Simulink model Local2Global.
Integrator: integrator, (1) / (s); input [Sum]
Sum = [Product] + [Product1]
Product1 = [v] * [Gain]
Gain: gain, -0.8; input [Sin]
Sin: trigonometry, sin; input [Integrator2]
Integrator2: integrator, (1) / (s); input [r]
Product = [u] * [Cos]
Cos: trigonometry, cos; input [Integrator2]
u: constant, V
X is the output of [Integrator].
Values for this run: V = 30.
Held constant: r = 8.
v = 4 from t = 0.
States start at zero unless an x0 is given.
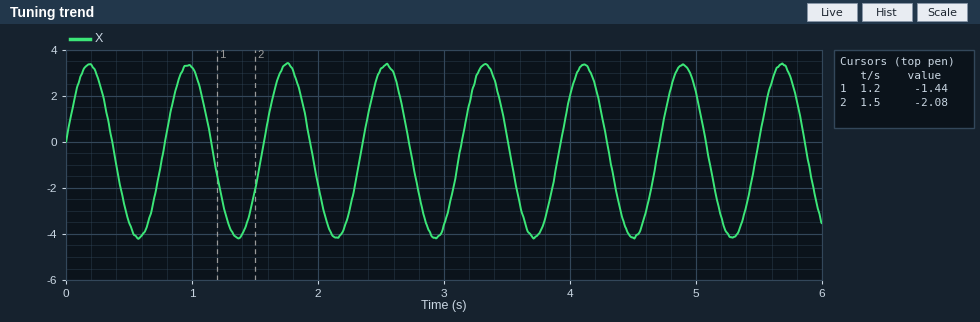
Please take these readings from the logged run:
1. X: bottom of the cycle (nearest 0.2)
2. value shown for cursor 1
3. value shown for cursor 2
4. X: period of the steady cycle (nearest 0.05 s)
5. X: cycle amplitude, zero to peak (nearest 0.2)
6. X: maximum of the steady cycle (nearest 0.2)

-4.2
-1.44
-2.08
0.80 s
3.8
3.4
